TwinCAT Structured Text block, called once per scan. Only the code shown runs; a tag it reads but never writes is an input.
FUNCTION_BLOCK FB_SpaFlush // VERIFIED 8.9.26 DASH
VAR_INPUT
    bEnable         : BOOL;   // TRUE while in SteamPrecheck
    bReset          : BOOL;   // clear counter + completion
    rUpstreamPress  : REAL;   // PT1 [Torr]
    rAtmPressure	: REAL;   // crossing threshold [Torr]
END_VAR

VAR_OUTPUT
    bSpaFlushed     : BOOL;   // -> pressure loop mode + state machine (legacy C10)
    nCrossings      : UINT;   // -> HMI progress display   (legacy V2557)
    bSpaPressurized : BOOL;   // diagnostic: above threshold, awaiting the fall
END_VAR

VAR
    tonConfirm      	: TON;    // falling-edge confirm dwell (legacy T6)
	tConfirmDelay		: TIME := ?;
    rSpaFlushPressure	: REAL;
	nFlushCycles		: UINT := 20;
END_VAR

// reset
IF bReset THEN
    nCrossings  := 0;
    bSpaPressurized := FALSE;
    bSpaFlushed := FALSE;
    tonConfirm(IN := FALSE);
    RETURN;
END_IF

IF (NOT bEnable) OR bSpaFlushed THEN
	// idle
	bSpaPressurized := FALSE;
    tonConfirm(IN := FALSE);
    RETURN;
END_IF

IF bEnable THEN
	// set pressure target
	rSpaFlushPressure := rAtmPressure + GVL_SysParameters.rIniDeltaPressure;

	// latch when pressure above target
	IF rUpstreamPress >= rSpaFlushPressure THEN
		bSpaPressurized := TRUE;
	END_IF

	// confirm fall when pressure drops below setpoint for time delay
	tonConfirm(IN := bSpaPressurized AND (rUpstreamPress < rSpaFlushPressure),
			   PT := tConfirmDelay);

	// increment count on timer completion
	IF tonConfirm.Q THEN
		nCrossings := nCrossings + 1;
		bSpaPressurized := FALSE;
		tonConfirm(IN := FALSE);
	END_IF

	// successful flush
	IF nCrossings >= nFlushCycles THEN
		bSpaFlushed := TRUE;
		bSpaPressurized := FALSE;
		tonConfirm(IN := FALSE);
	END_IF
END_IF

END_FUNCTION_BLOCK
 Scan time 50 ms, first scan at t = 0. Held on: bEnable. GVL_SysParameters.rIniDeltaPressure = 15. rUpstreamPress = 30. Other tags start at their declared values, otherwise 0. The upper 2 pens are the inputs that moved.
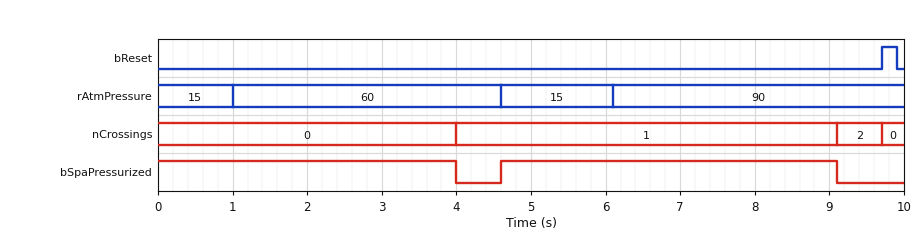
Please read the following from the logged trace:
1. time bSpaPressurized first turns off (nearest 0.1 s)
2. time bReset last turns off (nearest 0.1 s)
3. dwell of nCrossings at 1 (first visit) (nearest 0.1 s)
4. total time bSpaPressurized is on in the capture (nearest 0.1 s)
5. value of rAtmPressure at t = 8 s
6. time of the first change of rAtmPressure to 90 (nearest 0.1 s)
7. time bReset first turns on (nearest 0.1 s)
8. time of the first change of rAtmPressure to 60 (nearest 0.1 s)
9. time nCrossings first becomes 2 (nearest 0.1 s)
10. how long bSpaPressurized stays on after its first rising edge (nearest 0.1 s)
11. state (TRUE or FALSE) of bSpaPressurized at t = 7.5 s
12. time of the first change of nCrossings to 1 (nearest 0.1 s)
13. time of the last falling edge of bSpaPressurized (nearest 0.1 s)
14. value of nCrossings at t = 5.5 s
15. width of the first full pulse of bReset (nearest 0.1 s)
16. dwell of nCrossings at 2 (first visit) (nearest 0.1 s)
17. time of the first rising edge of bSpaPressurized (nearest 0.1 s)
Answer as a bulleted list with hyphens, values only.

- 4.0 s
- 9.9 s
- 5.1 s
- 8.5 s
- 90
- 6.1 s
- 9.7 s
- 1.0 s
- 9.1 s
- 4.5 s
- TRUE
- 4.0 s
- 9.1 s
- 1
- 0.2 s
- 0.6 s
- 4.6 s
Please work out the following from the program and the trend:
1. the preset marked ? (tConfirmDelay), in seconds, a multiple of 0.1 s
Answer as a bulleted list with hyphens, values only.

- 3.0 s
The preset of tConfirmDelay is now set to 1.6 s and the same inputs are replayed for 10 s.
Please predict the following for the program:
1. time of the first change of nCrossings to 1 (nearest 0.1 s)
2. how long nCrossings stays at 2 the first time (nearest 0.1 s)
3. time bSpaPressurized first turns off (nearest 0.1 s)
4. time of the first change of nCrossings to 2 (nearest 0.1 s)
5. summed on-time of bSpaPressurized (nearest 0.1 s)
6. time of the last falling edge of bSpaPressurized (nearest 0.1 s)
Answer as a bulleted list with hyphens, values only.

- 2.6 s
- 2.0 s
- 2.6 s
- 7.7 s
- 5.7 s
- 7.7 s
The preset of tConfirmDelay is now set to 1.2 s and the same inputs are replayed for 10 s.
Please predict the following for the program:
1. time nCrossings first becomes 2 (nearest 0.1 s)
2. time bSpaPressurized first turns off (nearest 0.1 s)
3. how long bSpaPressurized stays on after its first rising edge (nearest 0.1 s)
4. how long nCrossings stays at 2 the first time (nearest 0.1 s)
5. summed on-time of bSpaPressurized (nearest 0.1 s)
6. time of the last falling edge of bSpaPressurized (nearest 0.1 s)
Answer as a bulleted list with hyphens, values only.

- 7.3 s
- 2.2 s
- 2.7 s
- 2.4 s
- 4.9 s
- 7.3 s
